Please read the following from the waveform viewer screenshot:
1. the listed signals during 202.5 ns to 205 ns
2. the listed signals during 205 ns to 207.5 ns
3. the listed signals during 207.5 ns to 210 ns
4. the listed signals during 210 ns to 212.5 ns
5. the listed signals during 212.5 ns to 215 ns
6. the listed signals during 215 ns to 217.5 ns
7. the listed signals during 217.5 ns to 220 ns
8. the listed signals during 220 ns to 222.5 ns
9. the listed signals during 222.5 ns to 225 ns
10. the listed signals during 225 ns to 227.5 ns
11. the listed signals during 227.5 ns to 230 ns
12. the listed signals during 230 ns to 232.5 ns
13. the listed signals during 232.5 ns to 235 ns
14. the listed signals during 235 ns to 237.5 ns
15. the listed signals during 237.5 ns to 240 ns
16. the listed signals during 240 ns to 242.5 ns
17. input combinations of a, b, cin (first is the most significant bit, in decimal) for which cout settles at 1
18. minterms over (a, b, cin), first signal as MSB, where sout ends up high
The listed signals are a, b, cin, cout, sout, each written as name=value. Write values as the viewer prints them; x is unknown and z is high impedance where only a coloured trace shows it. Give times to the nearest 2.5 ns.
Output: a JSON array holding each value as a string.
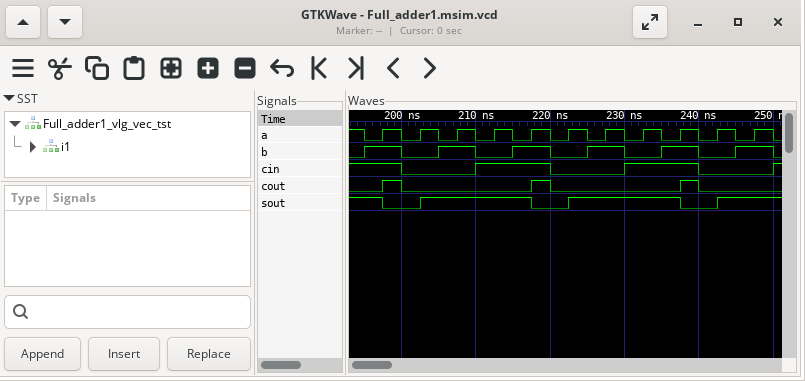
["a=1, b=0, cin=0, cout=0, sout=1", "a=0, b=1, cin=0, cout=0, sout=1", "a=1, b=1, cin=0, cout=0, sout=1", "a=0, b=0, cin=1, cout=0, sout=1", "a=1, b=0, cin=1, cout=0, sout=1", "a=0, b=1, cin=1, cout=0, sout=1", "a=1, b=1, cin=1, cout=1, sout=0", "a=0, b=0, cin=0, cout=0, sout=0", "a=1, b=0, cin=0, cout=0, sout=1", "a=0, b=1, cin=0, cout=0, sout=1", "a=1, b=1, cin=0, cout=0, sout=1", "a=0, b=0, cin=1, cout=0, sout=1", "a=1, b=0, cin=1, cout=0, sout=1", "a=0, b=1, cin=1, cout=0, sout=1", "a=1, b=1, cin=1, cout=1, sout=0", "a=0, b=0, cin=0, cout=0, sout=0", "7", "1, 2, 3, 4, 5, 6"]
